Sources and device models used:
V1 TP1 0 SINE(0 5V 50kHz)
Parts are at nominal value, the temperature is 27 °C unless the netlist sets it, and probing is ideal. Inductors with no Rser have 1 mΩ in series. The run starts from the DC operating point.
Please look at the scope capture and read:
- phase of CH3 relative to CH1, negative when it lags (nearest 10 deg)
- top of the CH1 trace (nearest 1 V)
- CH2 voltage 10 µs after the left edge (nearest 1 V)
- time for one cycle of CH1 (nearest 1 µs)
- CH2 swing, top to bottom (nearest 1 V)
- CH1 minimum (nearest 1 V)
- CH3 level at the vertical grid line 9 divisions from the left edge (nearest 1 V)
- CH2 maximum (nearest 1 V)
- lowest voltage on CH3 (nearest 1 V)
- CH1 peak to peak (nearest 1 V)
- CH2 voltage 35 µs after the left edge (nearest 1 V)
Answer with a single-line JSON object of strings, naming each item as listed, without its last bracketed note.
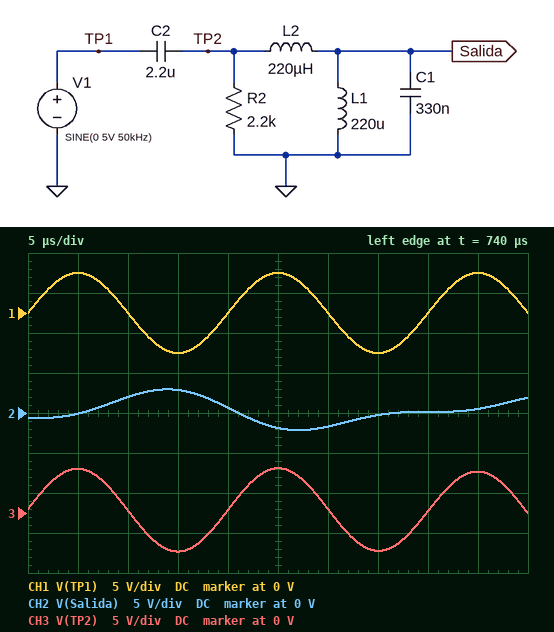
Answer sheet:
{"phase of CH3 relative to CH1, negative when it lags": "0 deg", "top of the CH1 trace": "5 V", "CH2 voltage 10 µs after the left edge": "2 V", "time for one cycle of CH1": "20 µs", "CH2 swing, top to bottom": "5 V", "CH1 minimum": "-5 V", "CH3 level at the vertical grid line 9 divisions from the left edge": "5 V", "CH2 maximum": "3 V", "lowest voltage on CH3": "-5 V", "CH1 peak to peak": "10 V", "CH2 voltage 35 µs after the left edge": "0 V"}
